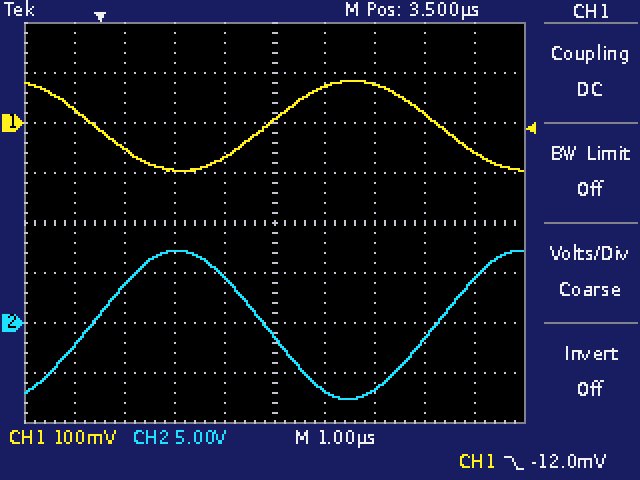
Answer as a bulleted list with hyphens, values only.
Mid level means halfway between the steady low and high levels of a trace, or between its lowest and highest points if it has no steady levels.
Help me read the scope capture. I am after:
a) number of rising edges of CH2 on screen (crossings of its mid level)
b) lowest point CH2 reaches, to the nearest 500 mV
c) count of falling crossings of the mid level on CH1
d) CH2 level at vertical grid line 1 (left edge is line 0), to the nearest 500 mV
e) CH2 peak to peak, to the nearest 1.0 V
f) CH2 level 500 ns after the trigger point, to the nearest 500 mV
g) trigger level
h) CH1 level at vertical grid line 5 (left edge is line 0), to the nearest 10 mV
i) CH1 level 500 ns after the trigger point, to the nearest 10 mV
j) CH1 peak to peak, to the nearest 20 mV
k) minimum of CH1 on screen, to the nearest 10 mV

- 2
- -7.5 V
- 2
- -2.5 V
- 15.0 V
- 4.0 V
- -12.0 mV
- 10 mV
- -50 mV
- 180 mV
- -100 mV
